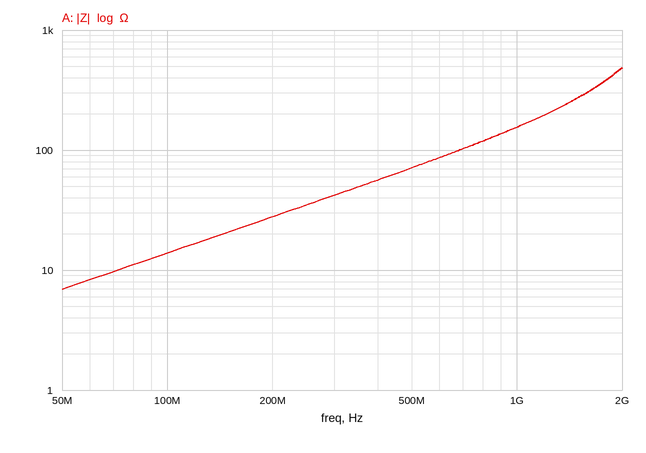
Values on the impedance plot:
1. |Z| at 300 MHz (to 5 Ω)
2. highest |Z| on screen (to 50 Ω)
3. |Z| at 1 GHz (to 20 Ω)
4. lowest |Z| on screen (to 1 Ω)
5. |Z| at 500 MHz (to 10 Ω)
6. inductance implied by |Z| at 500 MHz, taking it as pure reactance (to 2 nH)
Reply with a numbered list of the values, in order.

1. 40 Ω
2. 500 Ω
3. 160 Ω
4. 7 Ω
5. 70 Ω
6. 22 nH
